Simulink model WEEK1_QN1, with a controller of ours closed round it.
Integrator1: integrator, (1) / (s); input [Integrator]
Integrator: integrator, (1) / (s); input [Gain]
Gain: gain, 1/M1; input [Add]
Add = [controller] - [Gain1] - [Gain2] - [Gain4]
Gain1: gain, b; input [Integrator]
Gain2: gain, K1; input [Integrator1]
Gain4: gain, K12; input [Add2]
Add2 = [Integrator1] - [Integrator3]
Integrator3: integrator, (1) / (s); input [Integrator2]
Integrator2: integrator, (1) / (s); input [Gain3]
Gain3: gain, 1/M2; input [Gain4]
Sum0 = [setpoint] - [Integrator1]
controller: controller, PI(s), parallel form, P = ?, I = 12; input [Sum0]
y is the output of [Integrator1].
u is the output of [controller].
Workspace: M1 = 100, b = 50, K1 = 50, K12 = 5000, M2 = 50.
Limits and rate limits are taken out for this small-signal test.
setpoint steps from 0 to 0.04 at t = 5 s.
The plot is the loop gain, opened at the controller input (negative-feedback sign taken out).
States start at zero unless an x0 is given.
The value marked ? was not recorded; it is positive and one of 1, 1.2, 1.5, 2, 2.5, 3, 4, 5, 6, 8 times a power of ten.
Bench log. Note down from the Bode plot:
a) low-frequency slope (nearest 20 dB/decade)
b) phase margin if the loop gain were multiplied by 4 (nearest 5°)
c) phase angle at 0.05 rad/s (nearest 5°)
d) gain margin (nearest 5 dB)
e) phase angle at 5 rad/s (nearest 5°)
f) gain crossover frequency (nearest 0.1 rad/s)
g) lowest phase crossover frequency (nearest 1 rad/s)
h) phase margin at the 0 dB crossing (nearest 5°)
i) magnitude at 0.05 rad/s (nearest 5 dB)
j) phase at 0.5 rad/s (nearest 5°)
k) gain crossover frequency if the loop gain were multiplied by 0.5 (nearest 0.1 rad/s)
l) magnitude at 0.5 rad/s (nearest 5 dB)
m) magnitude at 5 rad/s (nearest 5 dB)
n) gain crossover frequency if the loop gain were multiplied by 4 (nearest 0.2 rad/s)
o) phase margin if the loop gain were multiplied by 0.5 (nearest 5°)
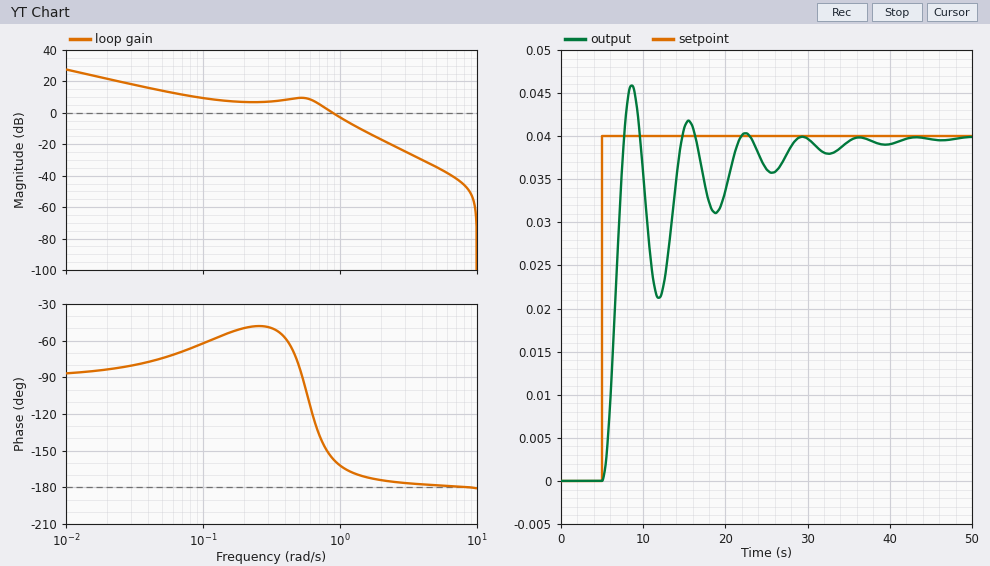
-20 dB/decade
10°
-75°
50 dB
-180°
0.9 rad/s
9 rad/s
25°
15 dB
-80°
0.7 rad/s
10 dB
-35 dB
1.6 rad/s
45°
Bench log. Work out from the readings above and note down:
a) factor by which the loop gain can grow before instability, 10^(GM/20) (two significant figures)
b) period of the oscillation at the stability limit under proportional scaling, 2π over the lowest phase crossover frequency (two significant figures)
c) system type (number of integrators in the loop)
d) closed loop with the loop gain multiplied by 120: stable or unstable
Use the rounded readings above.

320
0.70 s
1
stable
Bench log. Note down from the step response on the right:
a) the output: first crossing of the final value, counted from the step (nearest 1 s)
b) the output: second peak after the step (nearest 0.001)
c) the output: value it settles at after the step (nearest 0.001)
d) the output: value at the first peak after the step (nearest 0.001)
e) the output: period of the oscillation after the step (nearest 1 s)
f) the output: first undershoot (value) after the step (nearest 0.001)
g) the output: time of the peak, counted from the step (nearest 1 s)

3 s
0.042
0.040
0.046
7 s
0.021
4 s
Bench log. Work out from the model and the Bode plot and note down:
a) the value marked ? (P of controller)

80
